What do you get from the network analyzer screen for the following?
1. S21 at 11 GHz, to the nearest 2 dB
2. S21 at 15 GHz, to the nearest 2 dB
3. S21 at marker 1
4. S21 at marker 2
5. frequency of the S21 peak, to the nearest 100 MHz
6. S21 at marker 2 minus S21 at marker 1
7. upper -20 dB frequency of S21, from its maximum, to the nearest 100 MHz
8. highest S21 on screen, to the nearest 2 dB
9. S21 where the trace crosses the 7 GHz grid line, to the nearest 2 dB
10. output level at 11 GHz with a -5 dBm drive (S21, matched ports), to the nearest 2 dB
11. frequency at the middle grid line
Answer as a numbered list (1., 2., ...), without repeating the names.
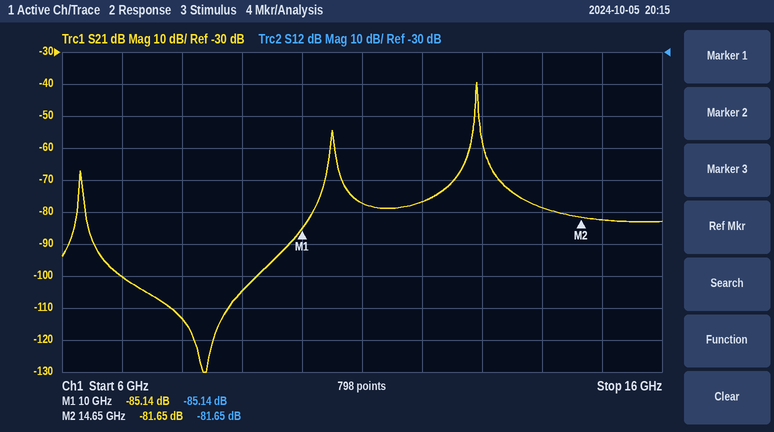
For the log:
1. -78 dB
2. -82 dB
3. -85.14 dB
4. -81.65 dB
5. 12.9 GHz
6. 3.49 dB
7. 13.0 GHz
8. -40 dB
9. -100 dB
10. -82 dBm
11. 11 GHz
